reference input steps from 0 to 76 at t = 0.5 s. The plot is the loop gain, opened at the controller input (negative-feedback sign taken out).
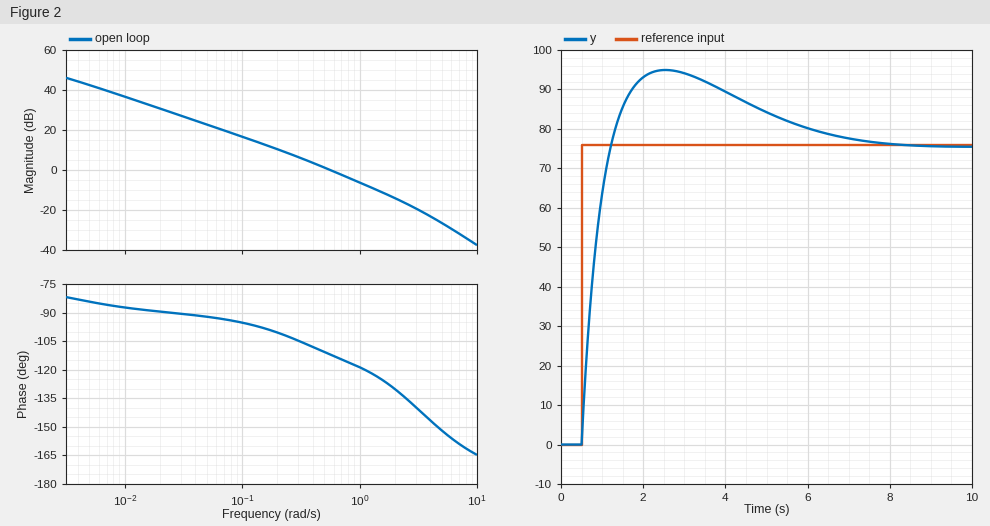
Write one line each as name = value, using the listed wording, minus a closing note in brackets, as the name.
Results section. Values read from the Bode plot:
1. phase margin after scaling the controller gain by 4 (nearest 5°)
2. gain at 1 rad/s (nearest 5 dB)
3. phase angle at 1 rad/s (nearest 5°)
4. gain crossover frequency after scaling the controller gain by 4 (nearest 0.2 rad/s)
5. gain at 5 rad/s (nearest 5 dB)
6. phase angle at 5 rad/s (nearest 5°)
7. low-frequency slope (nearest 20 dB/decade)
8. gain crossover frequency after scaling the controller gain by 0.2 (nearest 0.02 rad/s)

phase margin after scaling the controller gain by 4 = 55°
gain at 1 rad/s = -5 dB
phase angle at 1 rad/s = -120°
gain crossover frequency after scaling the controller gain by 4 = 1.6 rad/s
gain at 5 rad/s = -25 dB
phase angle at 5 rad/s = -150°
low-frequency slope = -20 dB/decade
gain crossover frequency after scaling the controller gain by 0.2 = 0.14 rad/s
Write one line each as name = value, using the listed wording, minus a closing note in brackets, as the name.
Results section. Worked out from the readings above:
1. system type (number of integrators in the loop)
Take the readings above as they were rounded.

system type = 1
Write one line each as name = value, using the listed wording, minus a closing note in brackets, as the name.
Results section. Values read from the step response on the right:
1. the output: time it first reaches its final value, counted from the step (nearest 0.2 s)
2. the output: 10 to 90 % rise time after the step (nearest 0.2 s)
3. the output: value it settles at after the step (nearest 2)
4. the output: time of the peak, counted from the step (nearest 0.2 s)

the output: time it first reaches its final value, counted from the step = 0.8 s
the output: 10 to 90 % rise time after the step = 0.6 s
the output: value it settles at after the step = 76
the output: time of the peak, counted from the step = 2.0 s
